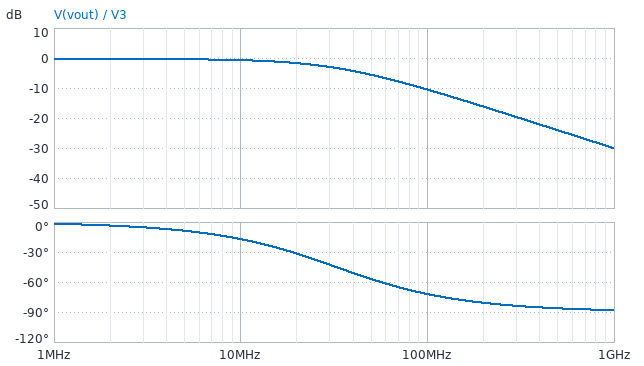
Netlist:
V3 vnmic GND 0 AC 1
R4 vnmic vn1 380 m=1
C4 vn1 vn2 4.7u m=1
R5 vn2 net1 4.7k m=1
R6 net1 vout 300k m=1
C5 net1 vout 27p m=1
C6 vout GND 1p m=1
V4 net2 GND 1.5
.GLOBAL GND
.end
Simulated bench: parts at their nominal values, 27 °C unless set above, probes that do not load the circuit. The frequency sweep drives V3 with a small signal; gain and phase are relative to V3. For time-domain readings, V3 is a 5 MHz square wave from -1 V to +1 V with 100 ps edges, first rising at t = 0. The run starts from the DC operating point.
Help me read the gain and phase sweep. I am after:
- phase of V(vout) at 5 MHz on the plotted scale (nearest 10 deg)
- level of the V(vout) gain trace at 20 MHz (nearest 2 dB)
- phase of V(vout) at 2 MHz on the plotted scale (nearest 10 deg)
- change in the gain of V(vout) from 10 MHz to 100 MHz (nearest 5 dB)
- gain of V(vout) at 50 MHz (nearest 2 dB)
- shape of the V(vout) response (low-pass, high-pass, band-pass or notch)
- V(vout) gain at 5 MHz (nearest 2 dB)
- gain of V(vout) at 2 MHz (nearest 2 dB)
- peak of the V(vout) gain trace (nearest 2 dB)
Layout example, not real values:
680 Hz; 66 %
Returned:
-10 deg; -2 dB; 0 deg; -10 dB; -6 dB; low-pass; 0 dB; 0 dB; 0 dB
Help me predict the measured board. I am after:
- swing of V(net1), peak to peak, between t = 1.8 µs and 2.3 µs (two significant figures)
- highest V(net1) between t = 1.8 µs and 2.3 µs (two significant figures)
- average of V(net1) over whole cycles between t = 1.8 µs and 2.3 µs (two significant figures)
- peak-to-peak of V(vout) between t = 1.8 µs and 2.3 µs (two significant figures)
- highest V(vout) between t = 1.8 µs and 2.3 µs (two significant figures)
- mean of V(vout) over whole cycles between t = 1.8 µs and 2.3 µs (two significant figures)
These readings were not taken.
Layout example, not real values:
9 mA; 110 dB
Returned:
2.0 V; 2.0 V; 1.0 V; 1.9 V; 1.9 V; 970 mV
